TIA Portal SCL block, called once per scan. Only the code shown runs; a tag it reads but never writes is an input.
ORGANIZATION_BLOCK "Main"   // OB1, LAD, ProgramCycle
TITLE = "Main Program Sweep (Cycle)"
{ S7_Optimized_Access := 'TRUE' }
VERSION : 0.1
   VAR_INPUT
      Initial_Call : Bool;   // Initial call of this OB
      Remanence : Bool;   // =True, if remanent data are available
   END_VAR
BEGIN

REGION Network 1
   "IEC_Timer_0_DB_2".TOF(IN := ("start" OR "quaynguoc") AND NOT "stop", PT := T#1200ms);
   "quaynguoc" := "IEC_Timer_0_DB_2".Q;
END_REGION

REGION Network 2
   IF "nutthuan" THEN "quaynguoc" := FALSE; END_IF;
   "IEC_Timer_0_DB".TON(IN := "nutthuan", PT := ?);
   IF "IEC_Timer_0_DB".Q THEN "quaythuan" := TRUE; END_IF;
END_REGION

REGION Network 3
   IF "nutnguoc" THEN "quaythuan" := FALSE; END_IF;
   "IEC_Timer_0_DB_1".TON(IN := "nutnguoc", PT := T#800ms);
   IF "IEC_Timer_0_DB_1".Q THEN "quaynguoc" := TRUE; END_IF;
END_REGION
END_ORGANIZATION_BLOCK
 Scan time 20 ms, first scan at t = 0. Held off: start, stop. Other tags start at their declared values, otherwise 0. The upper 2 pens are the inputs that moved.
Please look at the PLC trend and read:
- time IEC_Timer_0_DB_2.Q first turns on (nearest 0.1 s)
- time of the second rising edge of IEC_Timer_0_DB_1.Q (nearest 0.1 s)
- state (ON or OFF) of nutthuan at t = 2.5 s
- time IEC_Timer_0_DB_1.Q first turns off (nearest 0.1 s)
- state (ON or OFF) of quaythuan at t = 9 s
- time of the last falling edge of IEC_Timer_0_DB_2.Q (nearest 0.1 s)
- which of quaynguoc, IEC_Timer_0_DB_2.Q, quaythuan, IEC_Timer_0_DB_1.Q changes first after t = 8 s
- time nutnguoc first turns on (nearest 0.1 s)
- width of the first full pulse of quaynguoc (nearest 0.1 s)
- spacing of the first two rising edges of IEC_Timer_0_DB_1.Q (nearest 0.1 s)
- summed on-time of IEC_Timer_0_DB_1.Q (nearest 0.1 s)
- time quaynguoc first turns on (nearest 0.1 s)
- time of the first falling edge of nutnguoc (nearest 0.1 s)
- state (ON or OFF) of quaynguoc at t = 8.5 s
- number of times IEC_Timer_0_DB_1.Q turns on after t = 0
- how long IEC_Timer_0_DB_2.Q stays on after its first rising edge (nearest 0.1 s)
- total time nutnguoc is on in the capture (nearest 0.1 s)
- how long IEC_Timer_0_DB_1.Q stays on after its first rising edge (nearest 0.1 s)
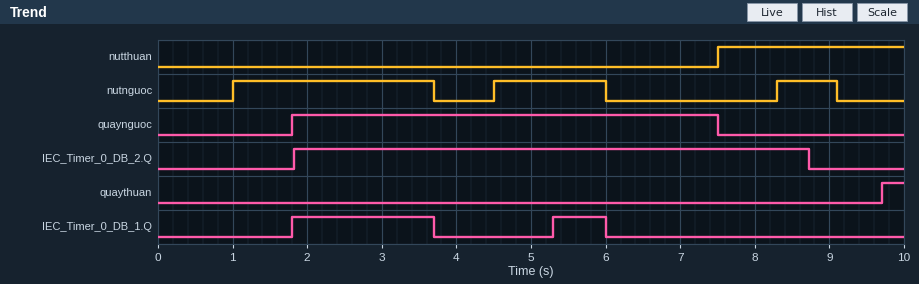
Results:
1.8 s
5.3 s
OFF
3.7 s
OFF
8.7 s
IEC_Timer_0_DB_2.Q
1.0 s
5.7 s
3.5 s
2.6 s
1.8 s
3.7 s
OFF
2
6.9 s
5.0 s
1.9 s
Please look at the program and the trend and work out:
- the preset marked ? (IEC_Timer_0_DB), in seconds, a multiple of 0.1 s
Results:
2.2 s
